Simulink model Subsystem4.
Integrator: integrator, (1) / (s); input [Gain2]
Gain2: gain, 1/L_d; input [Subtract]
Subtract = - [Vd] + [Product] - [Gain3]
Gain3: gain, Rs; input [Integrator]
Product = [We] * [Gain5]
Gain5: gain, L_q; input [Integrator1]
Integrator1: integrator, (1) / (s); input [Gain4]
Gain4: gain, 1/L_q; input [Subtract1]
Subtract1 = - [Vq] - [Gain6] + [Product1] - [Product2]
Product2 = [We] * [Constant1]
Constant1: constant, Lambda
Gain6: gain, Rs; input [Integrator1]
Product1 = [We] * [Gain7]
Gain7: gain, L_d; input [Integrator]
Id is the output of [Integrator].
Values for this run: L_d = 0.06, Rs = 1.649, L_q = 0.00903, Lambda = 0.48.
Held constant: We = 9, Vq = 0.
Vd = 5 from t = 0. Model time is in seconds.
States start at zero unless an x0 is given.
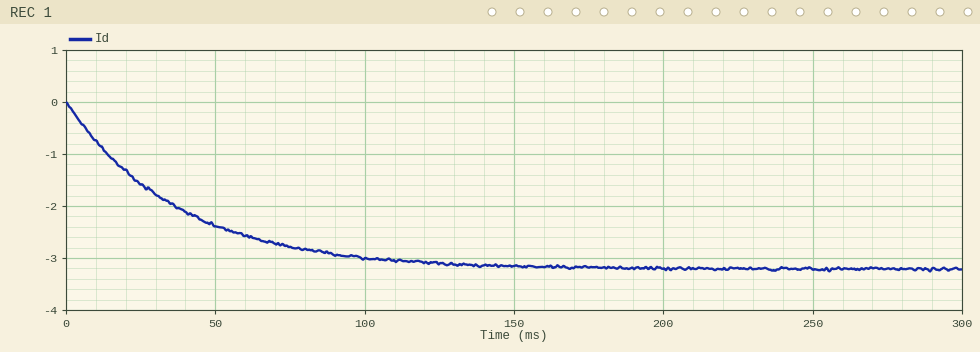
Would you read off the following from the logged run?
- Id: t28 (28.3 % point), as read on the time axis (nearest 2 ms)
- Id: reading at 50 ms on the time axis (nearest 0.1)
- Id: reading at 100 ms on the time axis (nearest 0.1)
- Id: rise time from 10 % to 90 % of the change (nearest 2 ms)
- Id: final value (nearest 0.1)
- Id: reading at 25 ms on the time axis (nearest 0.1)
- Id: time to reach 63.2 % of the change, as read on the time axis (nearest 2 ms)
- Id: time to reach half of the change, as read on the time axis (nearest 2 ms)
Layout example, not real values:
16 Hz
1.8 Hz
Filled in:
12 ms
-2.4
-3.0
82 ms
-3.2
-1.6
38 ms
26 ms
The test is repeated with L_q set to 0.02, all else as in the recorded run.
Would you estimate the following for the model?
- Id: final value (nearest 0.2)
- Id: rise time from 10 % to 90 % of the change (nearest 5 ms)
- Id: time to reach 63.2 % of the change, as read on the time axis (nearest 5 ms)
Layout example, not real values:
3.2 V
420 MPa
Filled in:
-3.4
85 ms
40 ms
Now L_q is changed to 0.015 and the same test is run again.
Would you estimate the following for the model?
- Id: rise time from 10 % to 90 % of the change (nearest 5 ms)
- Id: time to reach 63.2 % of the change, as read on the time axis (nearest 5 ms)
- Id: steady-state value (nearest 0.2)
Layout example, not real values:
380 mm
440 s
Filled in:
85 ms
40 ms
-3.4
